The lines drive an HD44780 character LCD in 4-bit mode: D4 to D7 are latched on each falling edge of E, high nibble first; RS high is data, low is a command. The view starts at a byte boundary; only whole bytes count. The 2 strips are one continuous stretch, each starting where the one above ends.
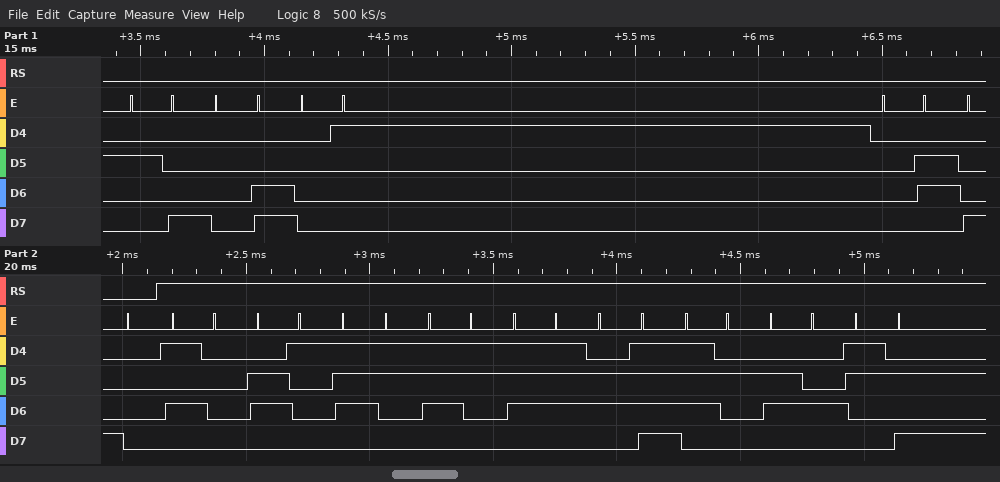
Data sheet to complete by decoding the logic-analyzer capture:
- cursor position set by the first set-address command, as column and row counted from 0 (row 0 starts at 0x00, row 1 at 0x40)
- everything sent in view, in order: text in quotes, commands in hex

column 0, row 0
0x28 0x0C 0x01 0x06 0x80 "Password:"
